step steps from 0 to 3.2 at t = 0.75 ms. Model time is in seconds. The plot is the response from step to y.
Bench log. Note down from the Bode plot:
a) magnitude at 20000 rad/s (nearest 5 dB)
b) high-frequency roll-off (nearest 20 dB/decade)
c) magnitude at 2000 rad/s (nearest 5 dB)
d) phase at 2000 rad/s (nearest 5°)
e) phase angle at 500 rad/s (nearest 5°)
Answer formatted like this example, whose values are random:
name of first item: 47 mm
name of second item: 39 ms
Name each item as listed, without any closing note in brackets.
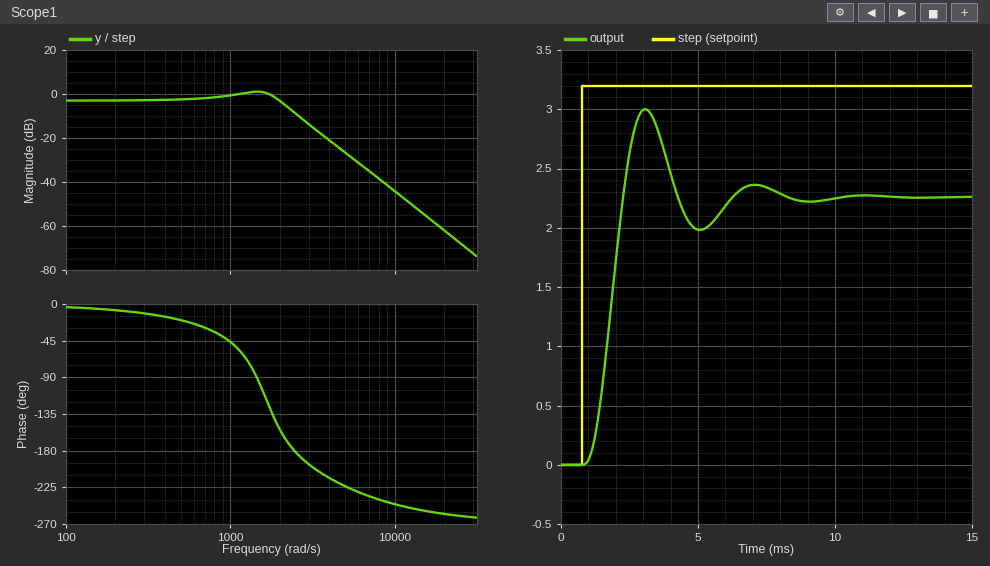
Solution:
magnitude at 20000 rad/s: -60 dB
high-frequency roll-off: -60 dB/decade
magnitude at 2000 rad/s: -5 dB
phase at 2000 rad/s: -155°
phase angle at 500 rad/s: -20°
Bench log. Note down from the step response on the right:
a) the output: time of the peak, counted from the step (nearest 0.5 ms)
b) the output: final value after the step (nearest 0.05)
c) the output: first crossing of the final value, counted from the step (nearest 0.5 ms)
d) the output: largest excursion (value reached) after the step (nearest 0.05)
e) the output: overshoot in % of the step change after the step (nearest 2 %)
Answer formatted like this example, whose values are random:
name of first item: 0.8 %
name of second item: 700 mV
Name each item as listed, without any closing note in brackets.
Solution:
the output: time of the peak, counted from the step: 2.5 ms
the output: final value after the step: 2.25
the output: first crossing of the final value, counted from the step: 1.5 ms
the output: largest excursion (value reached) after the step: 3.00
the output: overshoot in % of the step change after the step: 32 %
